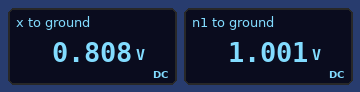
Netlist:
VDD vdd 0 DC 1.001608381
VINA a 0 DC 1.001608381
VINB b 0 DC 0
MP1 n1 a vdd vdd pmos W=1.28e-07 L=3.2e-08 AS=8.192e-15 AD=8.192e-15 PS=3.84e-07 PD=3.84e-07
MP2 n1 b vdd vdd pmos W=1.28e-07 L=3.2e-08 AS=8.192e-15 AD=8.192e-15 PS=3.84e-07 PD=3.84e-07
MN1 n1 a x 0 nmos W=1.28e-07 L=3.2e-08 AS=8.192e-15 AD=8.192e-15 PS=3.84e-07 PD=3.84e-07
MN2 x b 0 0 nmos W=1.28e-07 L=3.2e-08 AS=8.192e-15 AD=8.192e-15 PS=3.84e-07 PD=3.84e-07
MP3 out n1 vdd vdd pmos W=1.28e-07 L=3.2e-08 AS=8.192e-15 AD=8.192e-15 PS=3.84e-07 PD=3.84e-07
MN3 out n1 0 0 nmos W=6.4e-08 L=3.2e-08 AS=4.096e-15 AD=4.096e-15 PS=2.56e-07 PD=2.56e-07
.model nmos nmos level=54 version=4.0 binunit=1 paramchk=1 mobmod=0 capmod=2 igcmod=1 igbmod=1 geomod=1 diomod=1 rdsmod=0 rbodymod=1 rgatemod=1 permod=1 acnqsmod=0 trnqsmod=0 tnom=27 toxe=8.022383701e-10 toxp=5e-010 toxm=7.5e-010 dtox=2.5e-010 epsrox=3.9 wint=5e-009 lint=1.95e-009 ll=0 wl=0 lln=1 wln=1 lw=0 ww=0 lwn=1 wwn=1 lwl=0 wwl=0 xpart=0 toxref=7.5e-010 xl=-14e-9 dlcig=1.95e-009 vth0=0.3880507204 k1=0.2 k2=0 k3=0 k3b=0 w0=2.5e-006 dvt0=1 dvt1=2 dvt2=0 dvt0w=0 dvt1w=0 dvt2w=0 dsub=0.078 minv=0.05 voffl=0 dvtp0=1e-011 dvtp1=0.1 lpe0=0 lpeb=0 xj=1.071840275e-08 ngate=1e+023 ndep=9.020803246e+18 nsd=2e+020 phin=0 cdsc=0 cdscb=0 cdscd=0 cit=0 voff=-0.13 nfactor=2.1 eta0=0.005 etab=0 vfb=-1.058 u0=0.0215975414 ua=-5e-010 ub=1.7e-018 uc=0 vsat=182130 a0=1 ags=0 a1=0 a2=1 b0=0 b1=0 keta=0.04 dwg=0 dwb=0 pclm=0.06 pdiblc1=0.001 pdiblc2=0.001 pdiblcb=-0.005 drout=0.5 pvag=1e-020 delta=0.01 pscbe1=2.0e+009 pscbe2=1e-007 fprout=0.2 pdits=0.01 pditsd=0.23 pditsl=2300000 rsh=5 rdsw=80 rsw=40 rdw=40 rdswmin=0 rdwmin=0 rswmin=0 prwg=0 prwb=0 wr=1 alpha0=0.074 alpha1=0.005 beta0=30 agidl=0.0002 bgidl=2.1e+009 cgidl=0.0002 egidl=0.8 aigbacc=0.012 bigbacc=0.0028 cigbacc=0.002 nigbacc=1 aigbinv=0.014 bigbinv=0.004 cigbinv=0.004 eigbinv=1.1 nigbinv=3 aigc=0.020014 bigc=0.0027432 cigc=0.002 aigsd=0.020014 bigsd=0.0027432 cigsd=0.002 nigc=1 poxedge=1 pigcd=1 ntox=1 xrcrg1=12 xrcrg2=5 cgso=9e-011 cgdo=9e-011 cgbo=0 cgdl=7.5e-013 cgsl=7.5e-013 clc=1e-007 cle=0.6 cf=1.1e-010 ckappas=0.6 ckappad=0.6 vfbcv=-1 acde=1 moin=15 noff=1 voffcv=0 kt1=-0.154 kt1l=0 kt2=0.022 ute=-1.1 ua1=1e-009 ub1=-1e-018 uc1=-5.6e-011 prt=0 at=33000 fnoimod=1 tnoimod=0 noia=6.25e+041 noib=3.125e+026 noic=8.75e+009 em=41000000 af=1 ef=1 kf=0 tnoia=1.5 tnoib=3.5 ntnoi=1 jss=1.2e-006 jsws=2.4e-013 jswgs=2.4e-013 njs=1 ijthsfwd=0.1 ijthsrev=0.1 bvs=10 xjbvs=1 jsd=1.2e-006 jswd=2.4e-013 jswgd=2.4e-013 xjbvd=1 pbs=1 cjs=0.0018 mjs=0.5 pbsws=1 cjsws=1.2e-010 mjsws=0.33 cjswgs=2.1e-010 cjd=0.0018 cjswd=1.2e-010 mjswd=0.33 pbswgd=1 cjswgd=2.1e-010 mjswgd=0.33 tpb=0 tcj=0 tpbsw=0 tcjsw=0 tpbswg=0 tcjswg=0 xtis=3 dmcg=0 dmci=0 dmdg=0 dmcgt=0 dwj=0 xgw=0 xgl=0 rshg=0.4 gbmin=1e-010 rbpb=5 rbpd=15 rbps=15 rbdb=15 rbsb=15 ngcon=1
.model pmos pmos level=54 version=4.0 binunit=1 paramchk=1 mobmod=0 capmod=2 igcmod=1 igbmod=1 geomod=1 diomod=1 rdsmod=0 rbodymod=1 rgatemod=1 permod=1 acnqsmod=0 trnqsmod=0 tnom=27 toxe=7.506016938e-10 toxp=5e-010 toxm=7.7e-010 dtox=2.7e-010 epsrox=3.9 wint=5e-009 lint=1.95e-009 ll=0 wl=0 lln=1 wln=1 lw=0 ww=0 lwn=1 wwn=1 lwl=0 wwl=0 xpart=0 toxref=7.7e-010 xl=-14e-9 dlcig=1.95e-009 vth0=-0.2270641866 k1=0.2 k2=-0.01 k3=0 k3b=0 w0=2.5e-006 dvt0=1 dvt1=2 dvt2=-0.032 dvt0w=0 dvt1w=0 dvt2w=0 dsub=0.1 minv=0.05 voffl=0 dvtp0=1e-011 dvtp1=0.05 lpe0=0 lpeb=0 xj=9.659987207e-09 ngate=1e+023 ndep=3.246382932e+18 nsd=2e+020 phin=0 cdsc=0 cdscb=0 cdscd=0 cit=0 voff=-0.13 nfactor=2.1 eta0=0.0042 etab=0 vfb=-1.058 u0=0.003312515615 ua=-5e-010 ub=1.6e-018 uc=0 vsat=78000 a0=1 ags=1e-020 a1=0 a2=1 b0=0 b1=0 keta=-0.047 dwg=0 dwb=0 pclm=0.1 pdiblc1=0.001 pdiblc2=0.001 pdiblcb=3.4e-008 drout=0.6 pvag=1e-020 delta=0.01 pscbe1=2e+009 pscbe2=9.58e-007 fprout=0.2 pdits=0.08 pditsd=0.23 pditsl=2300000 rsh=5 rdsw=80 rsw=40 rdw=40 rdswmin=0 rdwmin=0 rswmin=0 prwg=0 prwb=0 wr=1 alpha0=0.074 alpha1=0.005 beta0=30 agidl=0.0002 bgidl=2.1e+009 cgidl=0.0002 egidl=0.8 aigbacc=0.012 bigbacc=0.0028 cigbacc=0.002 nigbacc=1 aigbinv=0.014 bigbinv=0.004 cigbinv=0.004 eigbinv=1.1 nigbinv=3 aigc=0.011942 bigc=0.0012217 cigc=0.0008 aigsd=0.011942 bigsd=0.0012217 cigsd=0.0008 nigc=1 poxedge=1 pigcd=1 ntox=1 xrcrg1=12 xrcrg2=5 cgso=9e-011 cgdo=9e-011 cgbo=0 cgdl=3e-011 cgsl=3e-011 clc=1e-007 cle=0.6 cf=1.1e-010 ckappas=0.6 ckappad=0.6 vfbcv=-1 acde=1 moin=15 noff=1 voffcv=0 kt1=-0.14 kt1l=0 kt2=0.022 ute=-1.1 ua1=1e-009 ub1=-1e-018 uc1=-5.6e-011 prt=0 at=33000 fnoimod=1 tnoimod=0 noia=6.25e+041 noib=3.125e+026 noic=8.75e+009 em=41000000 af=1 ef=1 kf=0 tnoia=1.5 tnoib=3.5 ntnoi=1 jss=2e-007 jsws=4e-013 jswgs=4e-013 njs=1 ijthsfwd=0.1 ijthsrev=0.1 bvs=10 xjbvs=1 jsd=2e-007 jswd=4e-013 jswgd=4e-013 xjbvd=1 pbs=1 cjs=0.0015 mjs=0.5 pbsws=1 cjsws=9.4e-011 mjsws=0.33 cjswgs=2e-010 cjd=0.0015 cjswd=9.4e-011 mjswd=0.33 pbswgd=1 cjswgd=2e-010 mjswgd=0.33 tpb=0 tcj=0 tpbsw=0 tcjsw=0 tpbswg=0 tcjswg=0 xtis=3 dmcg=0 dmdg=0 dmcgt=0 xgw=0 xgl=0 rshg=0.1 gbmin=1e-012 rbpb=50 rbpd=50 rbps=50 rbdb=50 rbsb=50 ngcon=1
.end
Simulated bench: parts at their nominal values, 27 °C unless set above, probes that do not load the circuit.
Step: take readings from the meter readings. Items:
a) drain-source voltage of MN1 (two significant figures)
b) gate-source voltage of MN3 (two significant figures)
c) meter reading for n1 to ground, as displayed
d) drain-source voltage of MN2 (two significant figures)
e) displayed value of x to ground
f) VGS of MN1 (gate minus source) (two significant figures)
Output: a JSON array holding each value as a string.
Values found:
["190 mV", "1.0 V", "1.001 V", "810 mV", "0.808 V", "190 mV"]
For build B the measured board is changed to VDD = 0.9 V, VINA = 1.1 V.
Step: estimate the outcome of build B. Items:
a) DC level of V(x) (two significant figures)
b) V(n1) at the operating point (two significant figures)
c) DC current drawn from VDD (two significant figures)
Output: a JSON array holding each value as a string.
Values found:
["860 mV", "900 mV", "170 nA"]
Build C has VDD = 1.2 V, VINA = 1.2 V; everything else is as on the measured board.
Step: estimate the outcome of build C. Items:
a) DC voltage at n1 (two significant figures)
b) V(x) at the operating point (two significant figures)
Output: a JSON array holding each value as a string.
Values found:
["1.2 V", "970 mV"]
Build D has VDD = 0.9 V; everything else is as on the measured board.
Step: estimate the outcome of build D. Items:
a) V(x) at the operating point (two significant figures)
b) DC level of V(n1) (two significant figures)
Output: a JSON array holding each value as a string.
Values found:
["800 mV", "900 mV"]
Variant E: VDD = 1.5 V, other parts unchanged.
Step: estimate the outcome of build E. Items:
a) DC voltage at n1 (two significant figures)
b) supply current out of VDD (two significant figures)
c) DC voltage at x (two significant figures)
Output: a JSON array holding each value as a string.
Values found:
["1.5 V", "9.1 µA", "860 mV"]
